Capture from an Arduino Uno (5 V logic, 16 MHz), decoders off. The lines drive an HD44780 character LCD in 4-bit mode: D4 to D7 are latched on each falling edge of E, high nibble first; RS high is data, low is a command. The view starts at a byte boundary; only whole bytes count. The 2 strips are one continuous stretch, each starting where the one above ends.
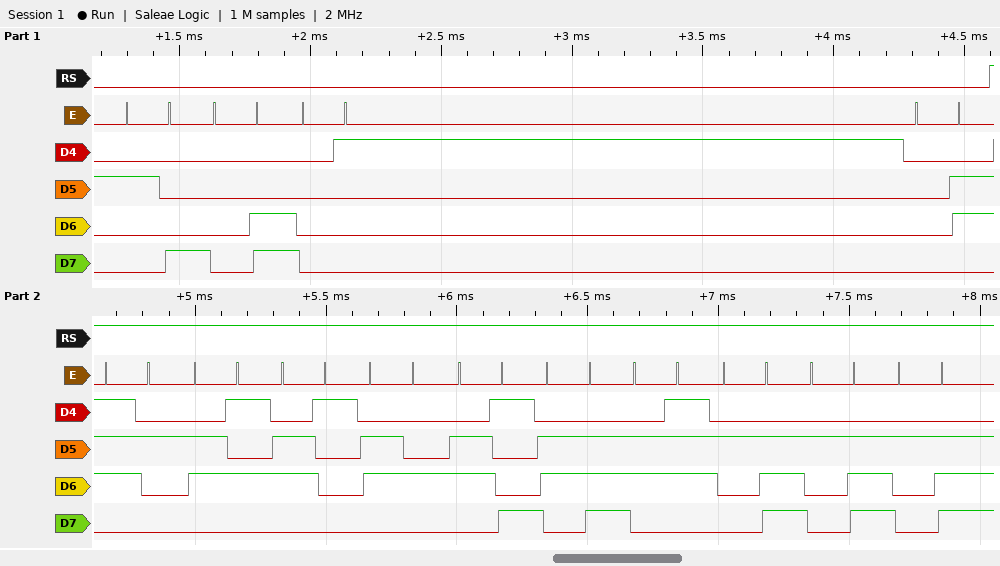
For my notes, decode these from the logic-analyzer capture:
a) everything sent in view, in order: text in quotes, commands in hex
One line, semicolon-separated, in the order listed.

0x28 0x0C 0x01 0x06 "reading..."
